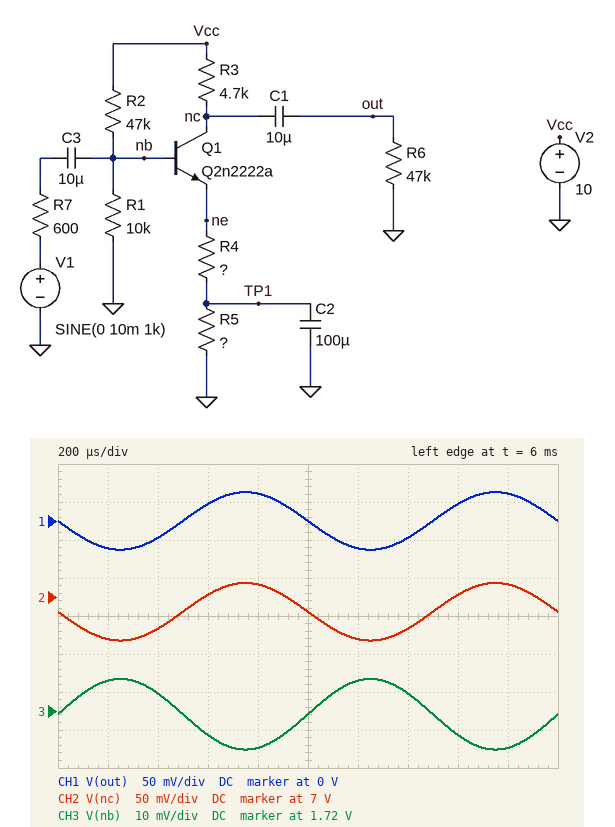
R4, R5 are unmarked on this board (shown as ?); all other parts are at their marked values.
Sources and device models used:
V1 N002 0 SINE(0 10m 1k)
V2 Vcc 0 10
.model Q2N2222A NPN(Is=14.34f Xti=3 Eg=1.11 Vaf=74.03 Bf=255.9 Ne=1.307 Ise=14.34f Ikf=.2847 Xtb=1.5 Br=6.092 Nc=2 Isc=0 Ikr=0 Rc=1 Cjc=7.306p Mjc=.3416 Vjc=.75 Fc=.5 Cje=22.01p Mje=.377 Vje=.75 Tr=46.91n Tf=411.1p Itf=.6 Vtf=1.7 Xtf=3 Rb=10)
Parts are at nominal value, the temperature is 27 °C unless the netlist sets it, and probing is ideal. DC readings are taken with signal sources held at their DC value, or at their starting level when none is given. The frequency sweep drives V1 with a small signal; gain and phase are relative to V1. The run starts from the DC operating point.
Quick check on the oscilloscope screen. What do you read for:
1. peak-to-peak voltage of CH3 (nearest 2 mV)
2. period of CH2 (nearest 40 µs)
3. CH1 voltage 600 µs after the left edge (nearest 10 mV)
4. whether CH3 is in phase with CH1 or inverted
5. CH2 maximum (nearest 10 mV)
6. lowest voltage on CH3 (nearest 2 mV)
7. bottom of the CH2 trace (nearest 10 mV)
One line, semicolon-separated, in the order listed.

18 mV; 1.00 ms; 20 mV; inverted; 7.02 V; 1.710 V; 6.94 V
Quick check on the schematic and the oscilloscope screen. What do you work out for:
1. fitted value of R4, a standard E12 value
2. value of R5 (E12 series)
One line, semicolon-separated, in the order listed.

1 kΩ; 680 Ω
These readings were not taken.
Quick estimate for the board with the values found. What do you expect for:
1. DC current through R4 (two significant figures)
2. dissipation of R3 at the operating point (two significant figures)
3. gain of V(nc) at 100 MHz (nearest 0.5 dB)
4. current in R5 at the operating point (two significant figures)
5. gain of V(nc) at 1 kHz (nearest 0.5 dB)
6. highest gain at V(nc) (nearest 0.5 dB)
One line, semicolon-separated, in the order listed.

650 µA; 1.9 mW; -3.5 dB; 650 µA; 11.5 dB; 11.5 dB
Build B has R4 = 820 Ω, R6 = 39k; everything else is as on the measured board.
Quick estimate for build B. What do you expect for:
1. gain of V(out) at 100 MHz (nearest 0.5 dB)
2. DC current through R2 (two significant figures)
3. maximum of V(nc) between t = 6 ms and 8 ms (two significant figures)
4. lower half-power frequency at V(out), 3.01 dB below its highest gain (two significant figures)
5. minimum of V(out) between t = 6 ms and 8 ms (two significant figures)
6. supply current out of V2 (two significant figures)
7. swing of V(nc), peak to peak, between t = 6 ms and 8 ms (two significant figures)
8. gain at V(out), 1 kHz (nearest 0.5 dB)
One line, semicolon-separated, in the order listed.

-4.0 dB; 180 µA; 6.7 V; 3.9 Hz; -45 mV; 890 µA; 90 mV; 13.0 dB
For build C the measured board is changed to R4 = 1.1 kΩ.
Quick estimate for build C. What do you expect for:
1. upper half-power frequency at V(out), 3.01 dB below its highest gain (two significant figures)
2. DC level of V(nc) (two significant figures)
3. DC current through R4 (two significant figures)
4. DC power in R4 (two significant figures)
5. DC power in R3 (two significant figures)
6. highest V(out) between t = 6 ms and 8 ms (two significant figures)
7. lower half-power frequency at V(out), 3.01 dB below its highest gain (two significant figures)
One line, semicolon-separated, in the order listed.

6.5 MHz; 7.1 V; 610 µA; 410 µW; 1.7 mW; 35 mV; 3.3 Hz
